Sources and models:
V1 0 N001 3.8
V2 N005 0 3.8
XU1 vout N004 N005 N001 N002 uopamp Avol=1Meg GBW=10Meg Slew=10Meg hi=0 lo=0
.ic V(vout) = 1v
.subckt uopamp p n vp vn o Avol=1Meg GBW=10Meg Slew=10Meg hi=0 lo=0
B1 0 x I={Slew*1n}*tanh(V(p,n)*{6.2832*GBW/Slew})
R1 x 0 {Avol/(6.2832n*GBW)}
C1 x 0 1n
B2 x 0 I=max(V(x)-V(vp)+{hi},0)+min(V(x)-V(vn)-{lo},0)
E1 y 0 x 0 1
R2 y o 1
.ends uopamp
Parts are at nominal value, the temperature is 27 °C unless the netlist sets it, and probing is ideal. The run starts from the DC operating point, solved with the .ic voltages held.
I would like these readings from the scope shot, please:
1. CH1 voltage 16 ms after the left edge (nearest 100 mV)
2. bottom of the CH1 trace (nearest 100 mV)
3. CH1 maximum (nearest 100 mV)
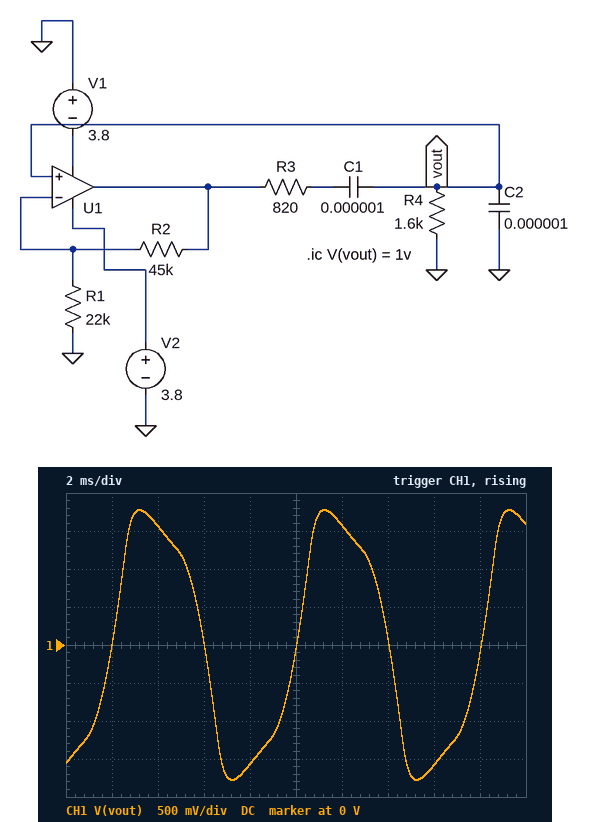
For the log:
-1.6 V
-1.8 V
1.8 V
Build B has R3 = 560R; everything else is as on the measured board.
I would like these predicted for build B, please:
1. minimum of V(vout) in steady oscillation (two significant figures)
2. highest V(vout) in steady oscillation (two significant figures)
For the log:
-2.0 V
2.0 V
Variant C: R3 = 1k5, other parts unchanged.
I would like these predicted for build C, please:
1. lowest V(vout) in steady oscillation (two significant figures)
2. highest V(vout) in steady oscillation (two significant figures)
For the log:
-1.4 V
1.4 V
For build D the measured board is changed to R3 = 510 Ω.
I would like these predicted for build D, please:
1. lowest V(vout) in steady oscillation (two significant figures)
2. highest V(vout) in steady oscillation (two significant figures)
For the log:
-2.0 V
2.0 V
